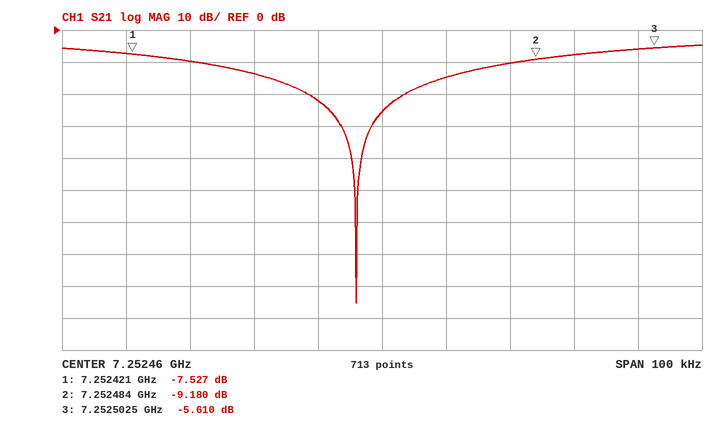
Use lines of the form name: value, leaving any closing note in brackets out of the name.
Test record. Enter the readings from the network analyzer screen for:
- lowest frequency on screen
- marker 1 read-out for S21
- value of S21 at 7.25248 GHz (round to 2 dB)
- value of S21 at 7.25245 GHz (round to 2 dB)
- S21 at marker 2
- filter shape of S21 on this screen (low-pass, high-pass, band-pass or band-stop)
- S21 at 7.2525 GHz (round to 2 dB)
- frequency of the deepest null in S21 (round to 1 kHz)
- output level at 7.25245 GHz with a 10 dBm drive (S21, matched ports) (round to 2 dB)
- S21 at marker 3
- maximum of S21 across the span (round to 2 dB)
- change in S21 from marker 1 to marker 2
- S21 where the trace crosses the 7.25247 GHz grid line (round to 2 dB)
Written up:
lowest frequency on screen: 7.25241 GHz
marker 1 read-out for S21: -7.527 dB
value of S21 at 7.25248 GHz: -10 dB
value of S21 at 7.25245 GHz: -22 dB
S21 at marker 2: -9.180 dB
filter shape of S21 on this screen: band-stop
S21 at 7.2525 GHz: -6 dB
frequency of the deepest null in S21: 7.252456 GHz
output level at 7.25245 GHz with a 10 dBm drive (S21, matched ports): -12 dBm
S21 at marker 3: -5.610 dB
maximum of S21 across the span: -4 dB
change in S21 from marker 1 to marker 2: -1.653 dB
S21 where the trace crosses the 7.25247 GHz grid line: -14 dB
